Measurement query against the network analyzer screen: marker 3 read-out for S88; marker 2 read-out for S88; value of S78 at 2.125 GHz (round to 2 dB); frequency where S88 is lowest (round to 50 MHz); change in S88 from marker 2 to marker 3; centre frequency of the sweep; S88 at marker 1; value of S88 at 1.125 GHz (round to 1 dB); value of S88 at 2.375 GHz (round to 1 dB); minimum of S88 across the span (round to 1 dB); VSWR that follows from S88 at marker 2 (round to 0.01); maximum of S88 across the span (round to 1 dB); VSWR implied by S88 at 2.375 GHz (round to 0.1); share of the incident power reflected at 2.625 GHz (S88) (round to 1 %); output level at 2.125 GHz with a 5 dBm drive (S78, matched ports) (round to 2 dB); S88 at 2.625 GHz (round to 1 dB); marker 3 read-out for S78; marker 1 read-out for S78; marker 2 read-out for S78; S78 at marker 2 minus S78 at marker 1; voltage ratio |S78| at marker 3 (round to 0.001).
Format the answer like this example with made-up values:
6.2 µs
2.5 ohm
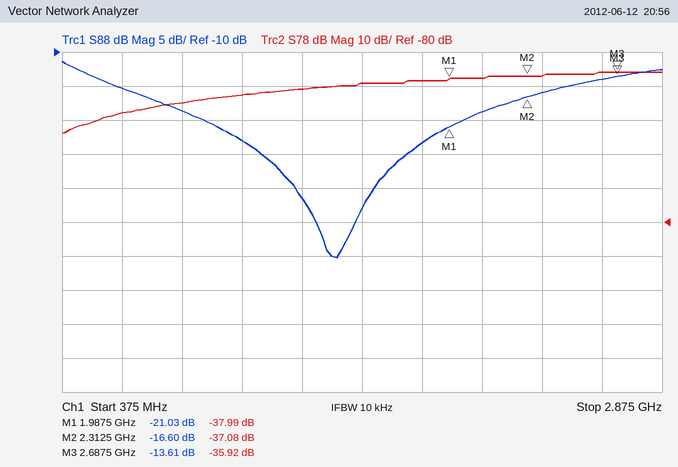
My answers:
-13.61 dB
-16.60 dB
-38 dB
1.50 GHz
2.99 dB
1.625 GHz
-21.03 dB
-23 dB
-16 dB
-40 dB
1.35
-11 dB
1.4
4 %
-32 dBm
-14 dB
-35.92 dB
-37.99 dB
-37.08 dB
0.91 dB
0.016
